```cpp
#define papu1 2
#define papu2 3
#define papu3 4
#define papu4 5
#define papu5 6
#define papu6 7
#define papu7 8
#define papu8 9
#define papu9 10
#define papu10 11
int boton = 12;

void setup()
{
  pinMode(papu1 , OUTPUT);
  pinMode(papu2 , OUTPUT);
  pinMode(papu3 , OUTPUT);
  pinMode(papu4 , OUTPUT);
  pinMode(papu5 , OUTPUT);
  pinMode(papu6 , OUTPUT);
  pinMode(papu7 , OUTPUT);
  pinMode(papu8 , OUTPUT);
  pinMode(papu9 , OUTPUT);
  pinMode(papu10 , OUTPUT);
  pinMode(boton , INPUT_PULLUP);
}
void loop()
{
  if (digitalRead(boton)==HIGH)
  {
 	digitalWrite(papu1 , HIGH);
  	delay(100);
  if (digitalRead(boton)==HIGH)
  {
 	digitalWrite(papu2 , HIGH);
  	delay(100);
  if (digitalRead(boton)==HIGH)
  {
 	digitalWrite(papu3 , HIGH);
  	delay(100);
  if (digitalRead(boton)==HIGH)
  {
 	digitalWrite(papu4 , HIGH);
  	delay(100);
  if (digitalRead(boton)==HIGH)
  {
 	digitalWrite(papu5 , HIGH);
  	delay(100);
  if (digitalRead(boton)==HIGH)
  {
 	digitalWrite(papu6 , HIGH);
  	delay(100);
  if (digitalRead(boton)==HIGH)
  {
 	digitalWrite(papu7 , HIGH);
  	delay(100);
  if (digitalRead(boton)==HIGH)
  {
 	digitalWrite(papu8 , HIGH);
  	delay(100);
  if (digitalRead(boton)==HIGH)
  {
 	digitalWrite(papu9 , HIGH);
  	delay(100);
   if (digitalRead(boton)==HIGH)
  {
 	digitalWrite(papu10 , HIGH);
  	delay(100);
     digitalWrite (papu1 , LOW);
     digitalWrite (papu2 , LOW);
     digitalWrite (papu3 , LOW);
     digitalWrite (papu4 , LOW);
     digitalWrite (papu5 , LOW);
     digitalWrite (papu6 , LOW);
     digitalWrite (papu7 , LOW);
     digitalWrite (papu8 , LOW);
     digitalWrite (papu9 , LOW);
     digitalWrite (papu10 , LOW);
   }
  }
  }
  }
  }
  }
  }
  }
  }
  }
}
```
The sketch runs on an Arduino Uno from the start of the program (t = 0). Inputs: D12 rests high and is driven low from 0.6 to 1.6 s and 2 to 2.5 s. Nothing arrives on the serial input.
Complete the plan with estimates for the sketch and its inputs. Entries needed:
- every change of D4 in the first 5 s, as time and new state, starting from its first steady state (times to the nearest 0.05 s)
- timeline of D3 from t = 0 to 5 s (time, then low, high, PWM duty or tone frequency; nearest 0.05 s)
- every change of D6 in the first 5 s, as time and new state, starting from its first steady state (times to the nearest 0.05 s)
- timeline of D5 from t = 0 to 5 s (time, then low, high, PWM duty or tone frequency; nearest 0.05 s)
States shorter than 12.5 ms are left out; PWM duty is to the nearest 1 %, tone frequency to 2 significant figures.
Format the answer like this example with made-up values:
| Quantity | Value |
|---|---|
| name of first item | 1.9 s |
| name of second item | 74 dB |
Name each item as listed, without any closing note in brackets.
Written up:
| Quantity | Value |
|---|---|
| every change of D4 in the first 5 s, as time and new state, starting from its first steady state | 0 s low; 0.2 s high; 3.5 s low; 3.7 s high; 4.5 s low; 4.7 s high |
| timeline of D3 from t = 0 to 5 s | 0 s low; 0.1 s high; 3.5 s low; 3.6 s high; 4.5 s low; 4.6 s high |
| every change of D6 in the first 5 s, as time and new state, starting from its first steady state | 0 s low; 0.4 s high; 3.5 s low; 3.9 s high; 4.5 s low; 4.9 s high |
| timeline of D5 from t = 0 to 5 s | 0 s low; 0.3 s high; 3.5 s low; 3.8 s high; 4.5 s low; 4.8 s high |
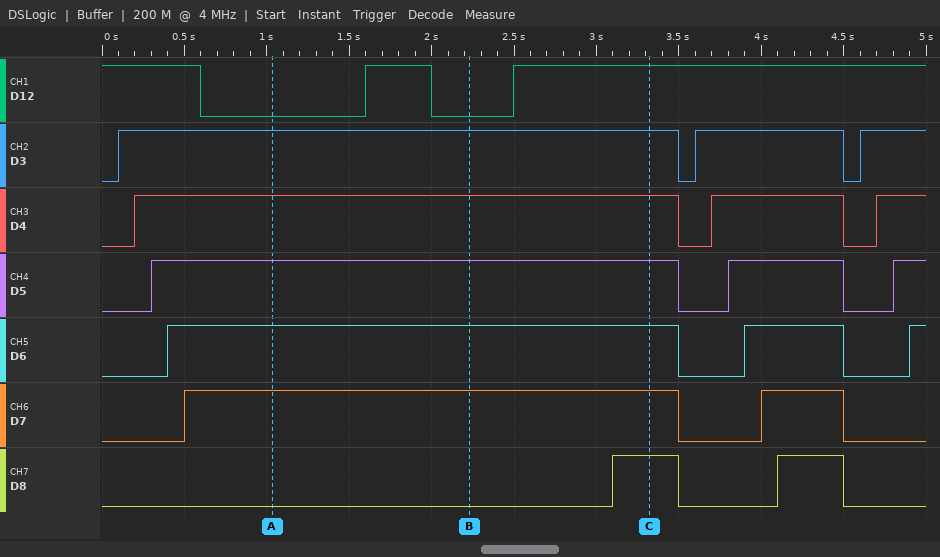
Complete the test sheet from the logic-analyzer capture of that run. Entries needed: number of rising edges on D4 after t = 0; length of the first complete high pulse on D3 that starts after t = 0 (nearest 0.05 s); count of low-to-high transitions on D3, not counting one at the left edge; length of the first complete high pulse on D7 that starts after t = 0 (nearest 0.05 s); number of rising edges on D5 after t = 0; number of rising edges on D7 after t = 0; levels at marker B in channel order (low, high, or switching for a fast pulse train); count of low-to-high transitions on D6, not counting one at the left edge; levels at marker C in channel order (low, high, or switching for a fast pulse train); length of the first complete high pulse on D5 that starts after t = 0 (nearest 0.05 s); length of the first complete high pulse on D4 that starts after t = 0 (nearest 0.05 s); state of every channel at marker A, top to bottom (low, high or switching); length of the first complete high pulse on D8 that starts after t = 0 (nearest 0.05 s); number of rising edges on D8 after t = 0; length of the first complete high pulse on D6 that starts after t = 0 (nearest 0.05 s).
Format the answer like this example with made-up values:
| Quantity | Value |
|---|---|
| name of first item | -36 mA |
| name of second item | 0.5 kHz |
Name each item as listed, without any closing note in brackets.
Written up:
| Quantity | Value |
|---|---|
| number of rising edges on D4 after t = 0 | 3 |
| length of the first complete high pulse on D3 that starts after t = 0 | 3.40 s |
| count of low-to-high transitions on D3, not counting one at the left edge | 3 |
| length of the first complete high pulse on D7 that starts after t = 0 | 3.00 s |
| number of rising edges on D5 after t = 0 | 3 |
| number of rising edges on D7 after t = 0 | 2 |
| levels at marker B in channel order | D12 low, D3 high, D4 high, D5 high, D6 high, D7 high, D8 low |
| count of low-to-high transitions on D6, not counting one at the left edge | 3 |
| levels at marker C in channel order | D12 high, D3 high, D4 high, D5 high, D6 high, D7 high, D8 high |
| length of the first complete high pulse on D5 that starts after t = 0 | 3.20 s |
| length of the first complete high pulse on D4 that starts after t = 0 | 3.30 s |
| state of every channel at marker A, top to bottom | D12 low, D3 high, D4 high, D5 high, D6 high, D7 high, D8 low |
| length of the first complete high pulse on D8 that starts after t = 0 | 0.40 s |
| number of rising edges on D8 after t = 0 | 2 |
| length of the first complete high pulse on D6 that starts after t = 0 | 3.10 s |
